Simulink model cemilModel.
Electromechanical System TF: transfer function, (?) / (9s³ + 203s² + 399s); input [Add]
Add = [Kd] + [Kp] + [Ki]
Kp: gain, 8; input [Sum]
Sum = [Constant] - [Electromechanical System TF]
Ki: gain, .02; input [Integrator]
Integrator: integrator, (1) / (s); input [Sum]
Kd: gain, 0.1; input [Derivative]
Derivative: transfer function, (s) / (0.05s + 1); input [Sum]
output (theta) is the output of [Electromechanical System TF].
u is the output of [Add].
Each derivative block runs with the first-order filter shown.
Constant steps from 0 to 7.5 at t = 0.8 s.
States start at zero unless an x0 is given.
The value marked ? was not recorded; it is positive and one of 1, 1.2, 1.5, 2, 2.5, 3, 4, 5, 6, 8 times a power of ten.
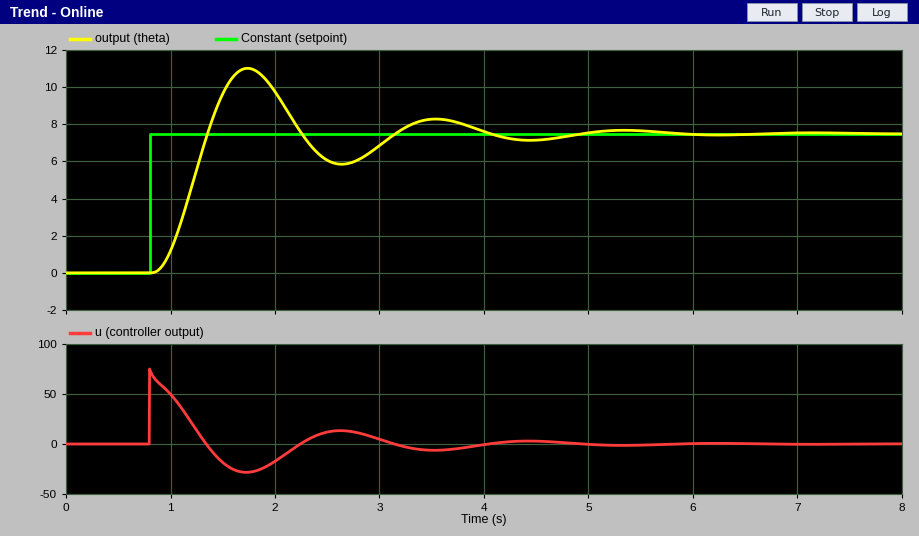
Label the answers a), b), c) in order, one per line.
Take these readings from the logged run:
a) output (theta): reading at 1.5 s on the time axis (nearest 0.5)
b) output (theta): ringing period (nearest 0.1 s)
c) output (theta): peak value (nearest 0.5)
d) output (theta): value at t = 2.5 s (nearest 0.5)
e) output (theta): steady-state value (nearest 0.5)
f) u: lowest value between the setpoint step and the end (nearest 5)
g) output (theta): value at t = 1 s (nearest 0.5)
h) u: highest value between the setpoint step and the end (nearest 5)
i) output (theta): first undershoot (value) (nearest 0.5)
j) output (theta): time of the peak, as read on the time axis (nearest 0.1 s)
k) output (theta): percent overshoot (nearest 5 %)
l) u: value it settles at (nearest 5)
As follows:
a) 9.5
b) 1.8 s
c) 11.0
d) 6.0
e) 7.5
f) -30
g) 1.0
h) 75
i) 6.0
j) 1.7 s
k) 45 %
l) 0
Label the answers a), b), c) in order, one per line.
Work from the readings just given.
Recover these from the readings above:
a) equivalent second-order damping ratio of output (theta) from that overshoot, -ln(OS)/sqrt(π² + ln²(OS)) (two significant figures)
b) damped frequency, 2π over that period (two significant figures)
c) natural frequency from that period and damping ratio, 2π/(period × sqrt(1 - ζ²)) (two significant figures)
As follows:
a) 0.25
b) 3.5 rad/s
c) 3.6 rad/s
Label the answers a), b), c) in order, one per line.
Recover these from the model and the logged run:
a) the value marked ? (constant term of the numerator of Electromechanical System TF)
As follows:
a) 300
